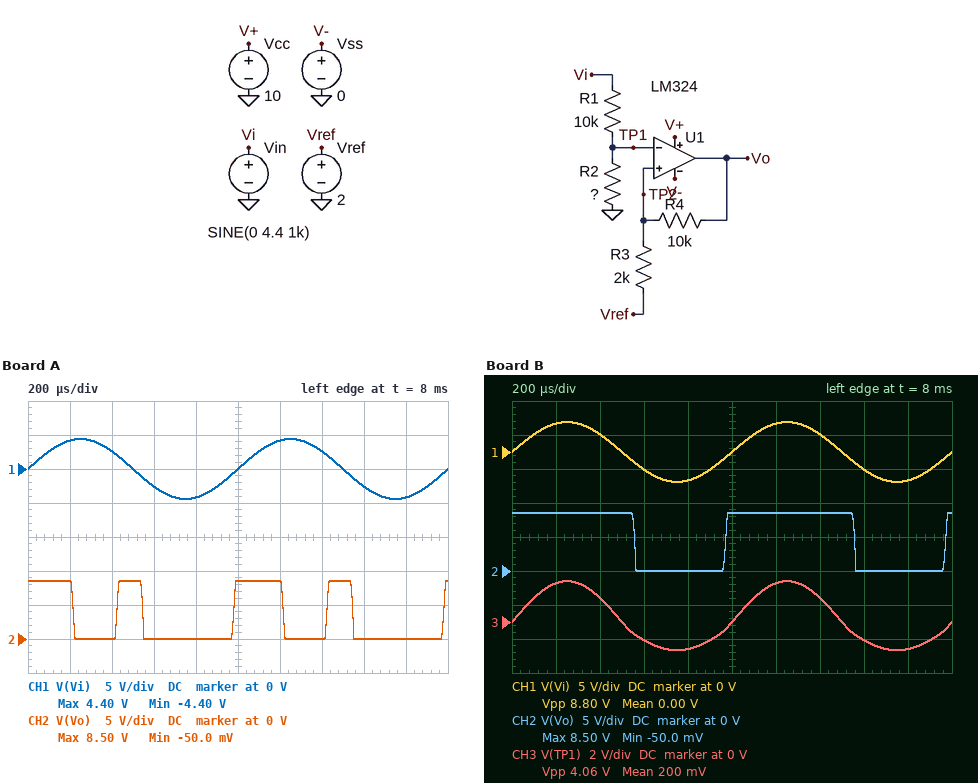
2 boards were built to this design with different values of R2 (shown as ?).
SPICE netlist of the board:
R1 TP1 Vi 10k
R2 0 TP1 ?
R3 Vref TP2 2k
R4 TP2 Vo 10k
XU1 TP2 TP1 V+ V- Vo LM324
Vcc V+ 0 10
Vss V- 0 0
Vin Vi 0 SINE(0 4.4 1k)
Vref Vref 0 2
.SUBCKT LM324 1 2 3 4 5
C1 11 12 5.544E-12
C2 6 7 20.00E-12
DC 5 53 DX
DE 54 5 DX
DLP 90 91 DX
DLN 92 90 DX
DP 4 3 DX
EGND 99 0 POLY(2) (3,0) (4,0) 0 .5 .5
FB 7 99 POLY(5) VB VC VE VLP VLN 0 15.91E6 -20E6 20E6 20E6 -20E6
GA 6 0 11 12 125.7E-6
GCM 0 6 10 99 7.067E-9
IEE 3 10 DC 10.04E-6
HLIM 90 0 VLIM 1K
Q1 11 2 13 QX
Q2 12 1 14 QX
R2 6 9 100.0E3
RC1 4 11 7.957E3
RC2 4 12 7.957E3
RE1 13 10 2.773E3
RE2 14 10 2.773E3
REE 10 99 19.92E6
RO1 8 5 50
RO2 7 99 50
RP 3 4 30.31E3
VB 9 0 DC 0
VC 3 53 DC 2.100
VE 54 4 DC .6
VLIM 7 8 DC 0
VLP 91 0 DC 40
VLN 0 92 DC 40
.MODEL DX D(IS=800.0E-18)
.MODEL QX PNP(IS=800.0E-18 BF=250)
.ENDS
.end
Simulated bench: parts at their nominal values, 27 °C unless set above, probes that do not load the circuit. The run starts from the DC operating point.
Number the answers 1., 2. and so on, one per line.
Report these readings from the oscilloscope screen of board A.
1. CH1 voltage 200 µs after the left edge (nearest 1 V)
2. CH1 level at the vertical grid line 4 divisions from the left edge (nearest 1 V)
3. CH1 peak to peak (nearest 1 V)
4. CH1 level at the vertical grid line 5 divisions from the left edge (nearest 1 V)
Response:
1. 4 V
2. -4 V
3. 9 V
4. 0 V
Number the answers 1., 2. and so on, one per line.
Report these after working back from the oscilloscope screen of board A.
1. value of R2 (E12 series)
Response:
1. 27 kΩ
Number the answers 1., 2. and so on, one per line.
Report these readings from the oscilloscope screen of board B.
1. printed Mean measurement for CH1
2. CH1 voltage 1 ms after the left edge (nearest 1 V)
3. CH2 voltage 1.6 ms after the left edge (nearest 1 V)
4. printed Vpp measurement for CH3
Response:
1. 0.00 V
2. 0 V
3. 0 V
4. 4.06 V
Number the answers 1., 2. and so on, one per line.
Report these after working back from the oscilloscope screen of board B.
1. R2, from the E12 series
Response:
1. 12 kΩ
